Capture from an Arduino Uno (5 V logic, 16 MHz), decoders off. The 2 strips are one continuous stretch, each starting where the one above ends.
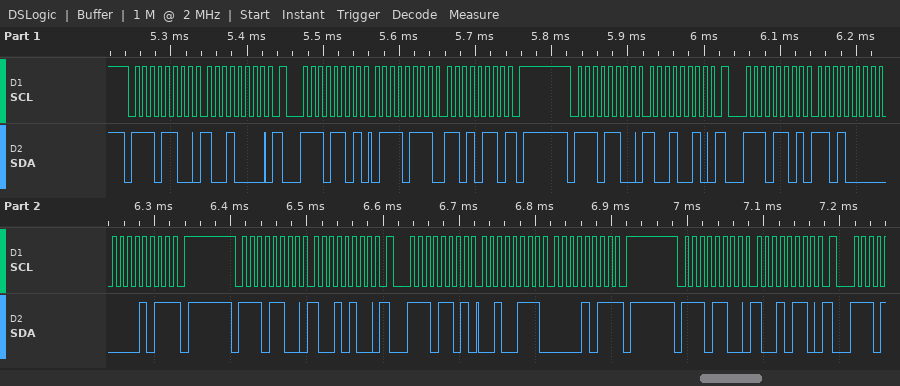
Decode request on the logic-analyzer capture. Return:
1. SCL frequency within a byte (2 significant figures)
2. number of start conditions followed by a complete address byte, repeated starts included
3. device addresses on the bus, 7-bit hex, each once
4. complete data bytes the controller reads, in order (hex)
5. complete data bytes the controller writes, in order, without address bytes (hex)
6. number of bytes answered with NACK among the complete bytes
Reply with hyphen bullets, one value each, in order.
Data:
- 100 kHz
- 7
- 0x76
- 77 D6 D0 0B 27 0B
- 90 92 94 96
- 3
